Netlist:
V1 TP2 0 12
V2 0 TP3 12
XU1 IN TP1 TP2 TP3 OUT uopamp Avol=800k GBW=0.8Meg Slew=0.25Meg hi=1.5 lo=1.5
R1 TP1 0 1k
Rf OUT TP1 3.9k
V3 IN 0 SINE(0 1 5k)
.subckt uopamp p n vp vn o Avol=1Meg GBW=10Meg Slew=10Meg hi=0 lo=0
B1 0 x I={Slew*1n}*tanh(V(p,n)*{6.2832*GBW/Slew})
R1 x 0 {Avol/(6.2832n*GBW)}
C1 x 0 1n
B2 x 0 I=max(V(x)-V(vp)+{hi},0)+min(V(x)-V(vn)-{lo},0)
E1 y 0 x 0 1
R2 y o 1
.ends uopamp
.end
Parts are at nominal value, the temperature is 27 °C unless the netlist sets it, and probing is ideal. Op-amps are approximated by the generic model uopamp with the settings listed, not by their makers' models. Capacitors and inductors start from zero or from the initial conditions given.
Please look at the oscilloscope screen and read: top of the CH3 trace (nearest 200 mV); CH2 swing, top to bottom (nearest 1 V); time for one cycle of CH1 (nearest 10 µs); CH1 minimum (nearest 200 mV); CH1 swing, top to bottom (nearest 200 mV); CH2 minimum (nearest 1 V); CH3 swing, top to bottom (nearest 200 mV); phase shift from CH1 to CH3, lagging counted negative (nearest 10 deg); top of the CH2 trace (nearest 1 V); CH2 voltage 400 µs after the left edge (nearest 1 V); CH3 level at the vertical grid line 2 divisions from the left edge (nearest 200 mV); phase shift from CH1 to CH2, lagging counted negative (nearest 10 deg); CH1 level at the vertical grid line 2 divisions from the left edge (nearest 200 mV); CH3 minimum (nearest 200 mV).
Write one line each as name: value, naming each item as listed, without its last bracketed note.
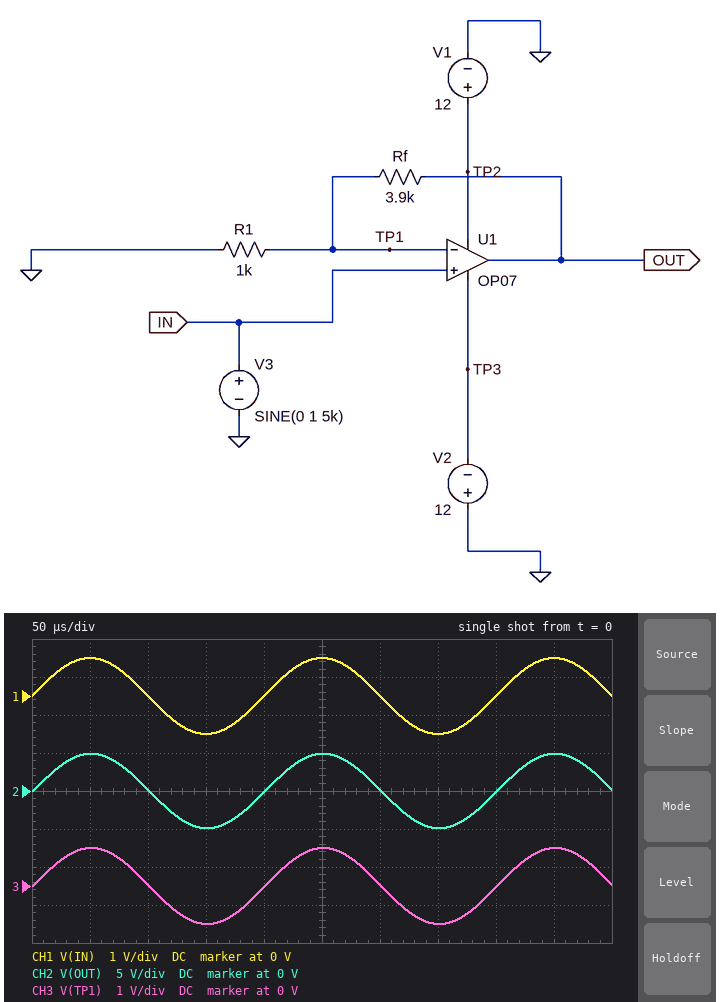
top of the CH3 trace: 1.0 V
CH2 swing, top to bottom: 10 V
time for one cycle of CH1: 200 µs
CH1 minimum: -1.0 V
CH1 swing, top to bottom: 2.0 V
CH2 minimum: -5 V
CH3 swing, top to bottom: 2.0 V
phase shift from CH1 to CH3, lagging counted negative: 0 deg
top of the CH2 trace: 5 V
CH2 voltage 400 µs after the left edge: 0 V
CH3 level at the vertical grid line 2 divisions from the left edge: 0 V
phase shift from CH1 to CH2, lagging counted negative: 0 deg
CH1 level at the vertical grid line 2 divisions from the left edge: 0 V
CH3 minimum: -1.0 V
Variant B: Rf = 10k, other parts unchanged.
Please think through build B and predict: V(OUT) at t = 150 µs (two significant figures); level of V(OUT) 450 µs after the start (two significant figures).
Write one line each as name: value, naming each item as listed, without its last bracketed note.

V(OUT) at t = 150 µs: -10 V
level of V(OUT) 450 µs after the start: 10 V
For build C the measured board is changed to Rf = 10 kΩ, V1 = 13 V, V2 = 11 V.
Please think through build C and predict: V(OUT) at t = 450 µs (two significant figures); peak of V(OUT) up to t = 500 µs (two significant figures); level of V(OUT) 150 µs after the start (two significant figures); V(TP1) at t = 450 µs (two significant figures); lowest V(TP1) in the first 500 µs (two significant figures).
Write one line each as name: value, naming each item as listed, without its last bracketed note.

V(OUT) at t = 450 µs: 10 V
peak of V(OUT) up to t = 500 µs: 11 V
level of V(OUT) 150 µs after the start: -9.5 V
V(TP1) at t = 450 µs: 920 mV
lowest V(TP1) in the first 500 µs: -860 mV
